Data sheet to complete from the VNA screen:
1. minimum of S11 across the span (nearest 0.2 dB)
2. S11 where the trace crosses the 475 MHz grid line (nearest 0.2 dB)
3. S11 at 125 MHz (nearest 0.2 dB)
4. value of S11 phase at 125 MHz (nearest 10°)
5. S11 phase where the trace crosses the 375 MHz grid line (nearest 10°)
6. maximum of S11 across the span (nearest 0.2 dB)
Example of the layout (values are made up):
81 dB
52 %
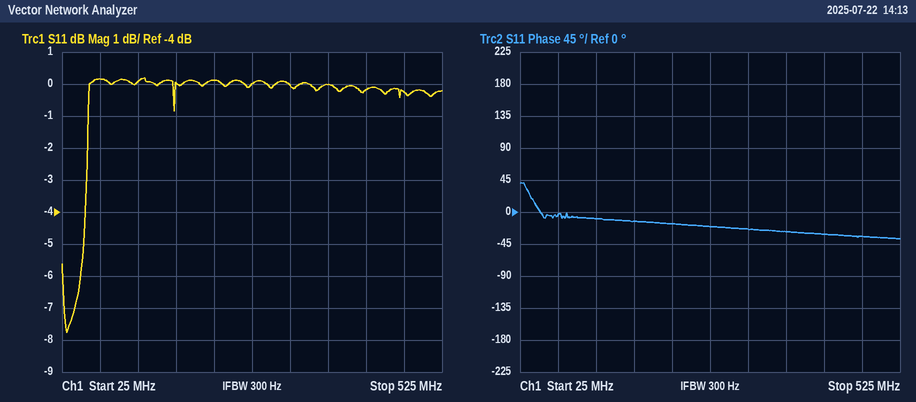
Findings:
-7.8 dB
-0.2 dB
0.0 dB
-10°
-30°
0.2 dB
